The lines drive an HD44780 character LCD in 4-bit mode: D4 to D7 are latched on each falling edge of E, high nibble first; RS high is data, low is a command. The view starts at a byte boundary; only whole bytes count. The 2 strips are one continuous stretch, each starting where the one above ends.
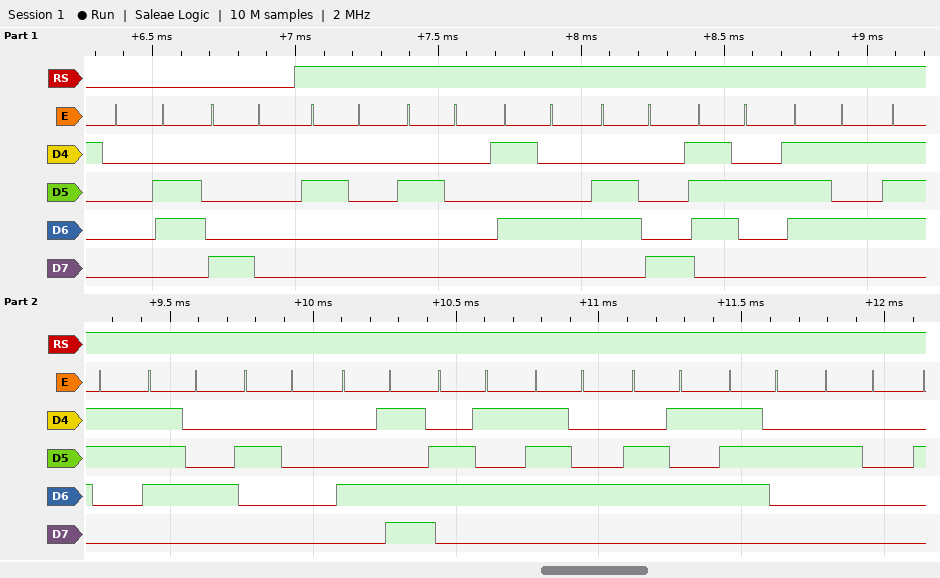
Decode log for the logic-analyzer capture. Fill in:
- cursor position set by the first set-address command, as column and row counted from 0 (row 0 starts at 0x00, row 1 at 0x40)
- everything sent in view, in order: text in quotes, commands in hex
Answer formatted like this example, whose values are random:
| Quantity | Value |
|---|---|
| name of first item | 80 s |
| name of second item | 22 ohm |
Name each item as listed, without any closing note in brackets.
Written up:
| Quantity | Value |
|---|---|
| cursor position set by the first set-address command, as column and row counted from 0 | column 0, row 0 |
| everything sent in view, in order: text in quotes, commands in hex | 0x06 0x80 "  Thrust Meter " |
